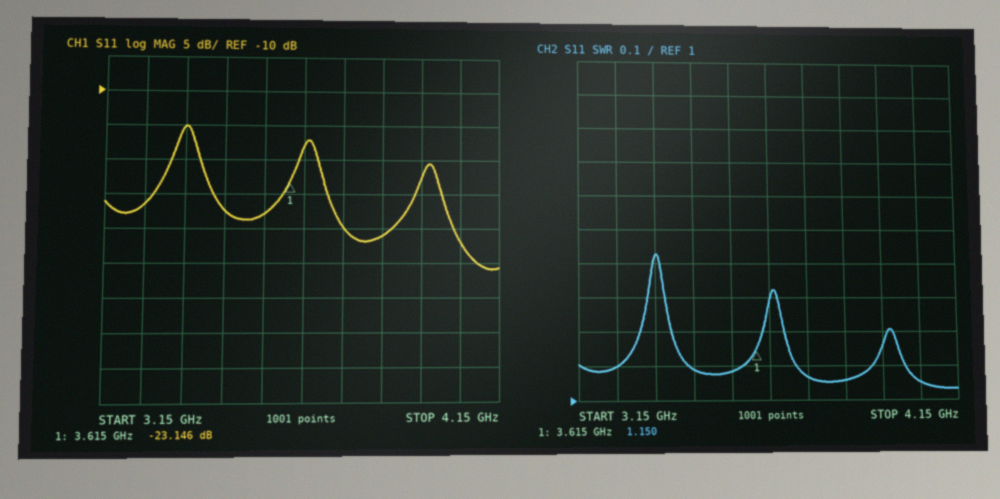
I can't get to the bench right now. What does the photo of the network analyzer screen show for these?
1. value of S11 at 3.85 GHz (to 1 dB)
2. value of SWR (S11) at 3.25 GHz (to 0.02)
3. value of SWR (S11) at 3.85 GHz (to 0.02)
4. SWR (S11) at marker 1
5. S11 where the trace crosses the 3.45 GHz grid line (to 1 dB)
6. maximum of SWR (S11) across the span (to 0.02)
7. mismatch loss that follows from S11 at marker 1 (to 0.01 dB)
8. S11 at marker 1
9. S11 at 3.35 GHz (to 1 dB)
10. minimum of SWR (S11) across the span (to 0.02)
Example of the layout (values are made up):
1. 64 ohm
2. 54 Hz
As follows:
1. -31 dB
2. 1.10
3. 1.06
4. 1.150
5. -27 dB
6. 1.42
7. 0.02 dB
8. -23.146 dB
9. -15 dB
10. 1.04
